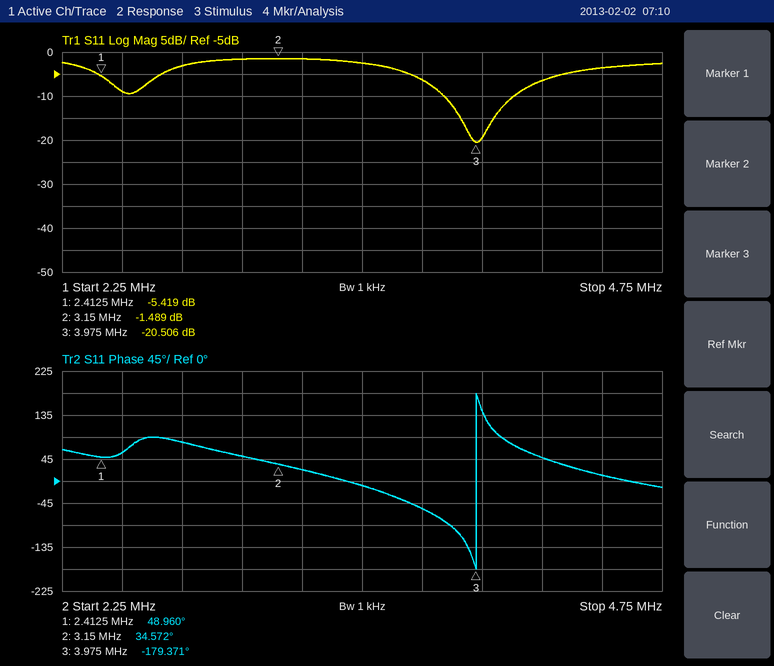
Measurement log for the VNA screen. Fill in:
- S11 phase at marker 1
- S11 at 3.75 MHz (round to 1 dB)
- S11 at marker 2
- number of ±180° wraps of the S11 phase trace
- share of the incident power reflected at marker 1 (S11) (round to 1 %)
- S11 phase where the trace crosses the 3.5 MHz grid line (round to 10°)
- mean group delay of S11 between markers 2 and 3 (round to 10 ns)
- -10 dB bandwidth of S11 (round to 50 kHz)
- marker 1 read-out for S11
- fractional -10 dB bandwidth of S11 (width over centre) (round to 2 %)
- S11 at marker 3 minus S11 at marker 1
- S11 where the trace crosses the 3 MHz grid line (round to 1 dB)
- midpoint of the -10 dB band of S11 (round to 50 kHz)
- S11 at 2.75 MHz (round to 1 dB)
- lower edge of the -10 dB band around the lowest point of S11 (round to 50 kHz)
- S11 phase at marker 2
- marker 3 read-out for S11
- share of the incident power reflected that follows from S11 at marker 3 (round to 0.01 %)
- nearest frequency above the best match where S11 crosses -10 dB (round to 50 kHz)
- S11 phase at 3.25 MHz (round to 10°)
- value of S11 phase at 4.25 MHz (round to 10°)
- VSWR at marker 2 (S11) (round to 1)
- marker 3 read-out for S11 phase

48.960°
-6 dB
-1.489 dB
1
29 %
-10°
720 ns
300 kHz
-5.419 dB
8 %
-15.087 dB
-2 dB
4.00 MHz
-3 dB
3.85 MHz
34.572°
-20.506 dB
0.89 %
4.15 MHz
20°
50°
12
-179.371°
